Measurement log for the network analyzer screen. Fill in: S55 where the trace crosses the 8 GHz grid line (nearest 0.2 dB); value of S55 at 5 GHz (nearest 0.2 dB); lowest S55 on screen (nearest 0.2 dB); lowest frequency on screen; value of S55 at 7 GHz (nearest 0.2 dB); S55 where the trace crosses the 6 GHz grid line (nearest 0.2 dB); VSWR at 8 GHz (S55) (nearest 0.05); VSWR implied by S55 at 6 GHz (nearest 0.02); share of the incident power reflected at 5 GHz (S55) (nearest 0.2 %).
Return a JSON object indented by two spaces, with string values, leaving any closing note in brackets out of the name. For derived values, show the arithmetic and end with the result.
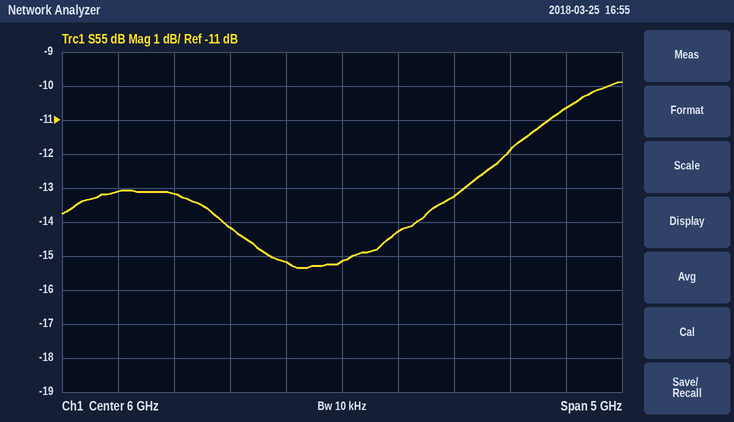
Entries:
{
  "S55 where the trace crosses the 8 GHz grid line": "-10.6 dB",
  "value of S55 at 5 GHz": "-14.2 dB",
  "lowest S55 on screen": "-15.4 dB",
  "lowest frequency on screen": "3.5 GHz",
  "value of S55 at 7 GHz": "-13.2 dB",
  "S55 where the trace crosses the 6 GHz grid line": "-15.2 dB",
  "VSWR at 8 GHz (S55)": "|Γ| = 10^(-10.6/20) = 0.2951; VSWR = (1 + 0.2951)/(1 − 0.2951) ≈ 1.84, so 1.85 to the nearest 0.05",
  "VSWR implied by S55 at 6 GHz": "|Γ| = 10^(-15.2/20) = 0.1738; VSWR = (1 + 0.1738)/(1 − 0.1738) ≈ 1.42",
  "share of the incident power reflected at 5 GHz (S55)": "10^(-14.2/10) ≈ 3.8 %"
}
